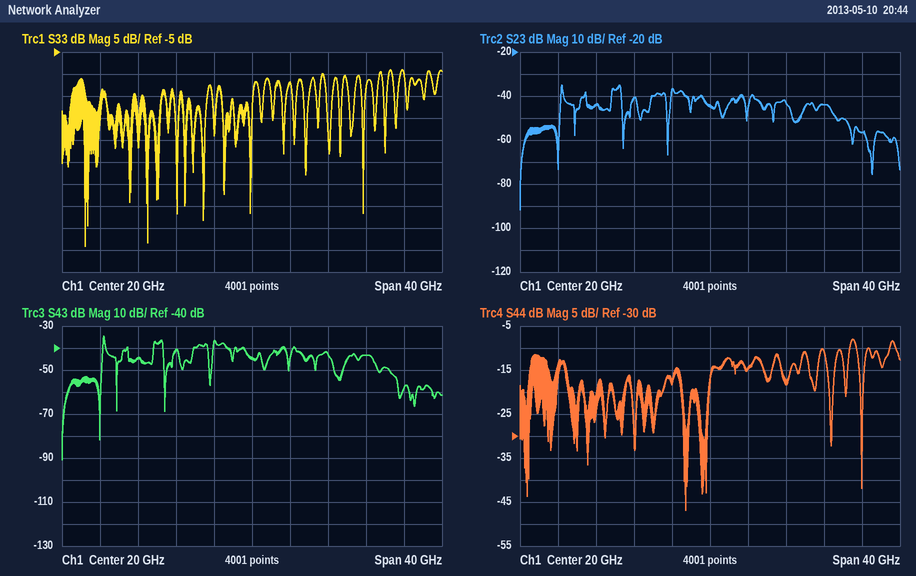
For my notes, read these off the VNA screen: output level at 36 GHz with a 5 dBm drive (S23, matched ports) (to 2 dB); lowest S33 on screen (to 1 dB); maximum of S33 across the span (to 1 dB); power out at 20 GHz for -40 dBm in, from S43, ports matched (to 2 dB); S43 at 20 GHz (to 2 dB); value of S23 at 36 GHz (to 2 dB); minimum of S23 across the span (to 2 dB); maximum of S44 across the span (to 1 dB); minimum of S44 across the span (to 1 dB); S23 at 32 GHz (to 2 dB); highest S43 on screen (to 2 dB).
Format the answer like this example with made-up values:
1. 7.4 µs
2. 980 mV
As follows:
1. -52 dBm
2. -49 dB
3. -9 dB
4. -84 dBm
5. -44 dB
6. -56 dB
7. -92 dB
8. -8 dB
9. -47 dB
10. -44 dB
11. -34 dB
